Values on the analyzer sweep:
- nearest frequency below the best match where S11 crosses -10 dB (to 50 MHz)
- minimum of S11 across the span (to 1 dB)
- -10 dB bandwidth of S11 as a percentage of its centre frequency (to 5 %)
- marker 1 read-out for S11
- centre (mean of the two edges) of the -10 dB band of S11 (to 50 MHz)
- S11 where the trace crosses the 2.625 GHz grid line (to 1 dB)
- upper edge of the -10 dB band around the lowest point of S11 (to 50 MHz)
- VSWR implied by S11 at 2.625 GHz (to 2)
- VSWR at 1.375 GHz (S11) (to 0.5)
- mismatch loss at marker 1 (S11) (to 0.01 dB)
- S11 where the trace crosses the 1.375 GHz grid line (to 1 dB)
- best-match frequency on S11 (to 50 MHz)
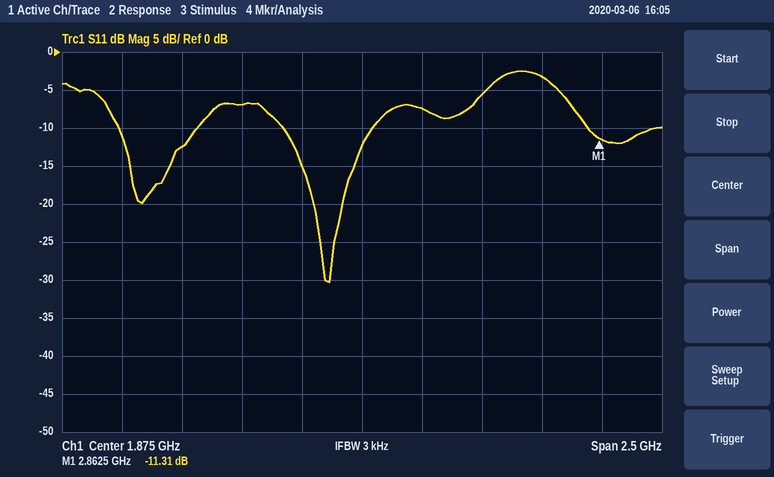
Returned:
1.55 GHz
-30 dB
20 %
-11.31 dB
1.75 GHz
-3 dB
1.90 GHz
6
2.5
0.33 dB
-7 dB
1.75 GHz
